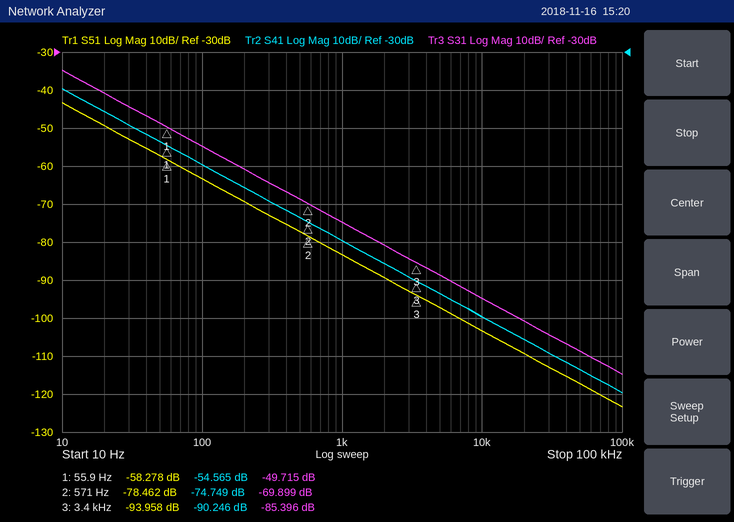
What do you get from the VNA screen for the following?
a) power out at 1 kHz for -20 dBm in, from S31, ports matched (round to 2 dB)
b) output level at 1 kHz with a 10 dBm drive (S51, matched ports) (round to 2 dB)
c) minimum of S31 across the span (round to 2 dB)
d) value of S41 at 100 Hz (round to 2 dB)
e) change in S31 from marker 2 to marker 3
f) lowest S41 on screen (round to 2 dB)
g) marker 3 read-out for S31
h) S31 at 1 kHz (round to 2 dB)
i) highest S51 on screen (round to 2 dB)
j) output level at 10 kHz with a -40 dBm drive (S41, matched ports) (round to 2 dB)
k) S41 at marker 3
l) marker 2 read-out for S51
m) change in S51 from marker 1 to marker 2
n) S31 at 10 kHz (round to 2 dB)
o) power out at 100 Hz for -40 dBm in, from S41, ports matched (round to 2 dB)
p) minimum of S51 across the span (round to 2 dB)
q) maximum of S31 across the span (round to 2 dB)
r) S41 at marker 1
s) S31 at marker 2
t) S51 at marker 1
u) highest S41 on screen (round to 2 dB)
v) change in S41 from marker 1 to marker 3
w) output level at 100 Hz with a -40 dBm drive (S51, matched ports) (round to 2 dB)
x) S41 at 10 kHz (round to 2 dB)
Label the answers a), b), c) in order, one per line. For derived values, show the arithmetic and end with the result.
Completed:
a) -20 dBm + (-74 dB) = -94 dBm
b) 10 dBm + (-84 dB) = -74 dBm
c) -114 dB
d) -60 dB
e) -85.396 − (-69.899) = -15.497 dB
f) -120 dB
g) -85.396 dB
h) -74 dB
i) -44 dB
j) -40 dBm + (-100 dB) = -140 dBm
k) -90.246 dB
l) -78.462 dB
m) -78.462 − (-58.278) = -20.184 dB
n) -94 dB
o) -40 dBm + (-60 dB) = -100 dBm
p) -124 dB
q) -34 dB
r) -54.565 dB
s) -69.899 dB
t) -58.278 dB
u) -40 dB
v) -90.246 − (-54.565) = -35.681 dB
w) -40 dBm + (-64 dB) = -104 dBm
x) -100 dB
